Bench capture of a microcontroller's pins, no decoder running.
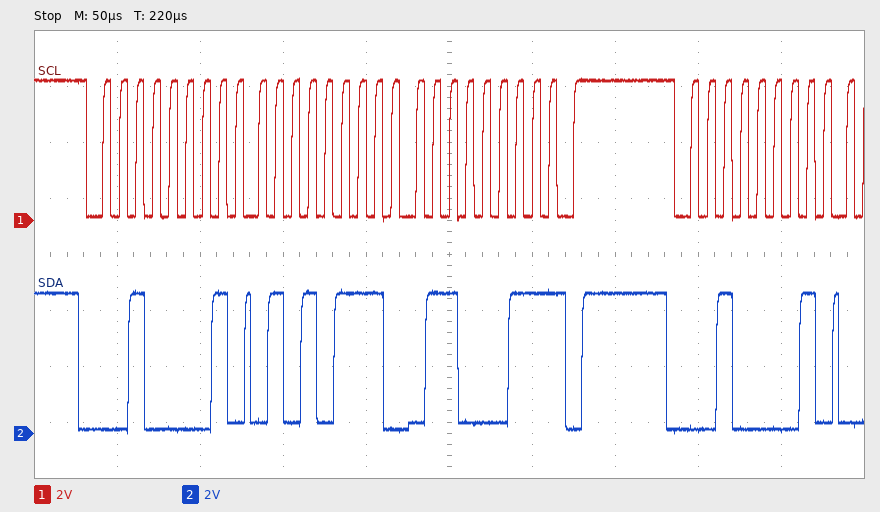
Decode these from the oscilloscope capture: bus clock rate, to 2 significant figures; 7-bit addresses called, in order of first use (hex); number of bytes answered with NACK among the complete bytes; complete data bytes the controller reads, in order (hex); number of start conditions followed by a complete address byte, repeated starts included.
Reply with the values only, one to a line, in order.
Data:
100 kHz
0x10
1
57 63
2
